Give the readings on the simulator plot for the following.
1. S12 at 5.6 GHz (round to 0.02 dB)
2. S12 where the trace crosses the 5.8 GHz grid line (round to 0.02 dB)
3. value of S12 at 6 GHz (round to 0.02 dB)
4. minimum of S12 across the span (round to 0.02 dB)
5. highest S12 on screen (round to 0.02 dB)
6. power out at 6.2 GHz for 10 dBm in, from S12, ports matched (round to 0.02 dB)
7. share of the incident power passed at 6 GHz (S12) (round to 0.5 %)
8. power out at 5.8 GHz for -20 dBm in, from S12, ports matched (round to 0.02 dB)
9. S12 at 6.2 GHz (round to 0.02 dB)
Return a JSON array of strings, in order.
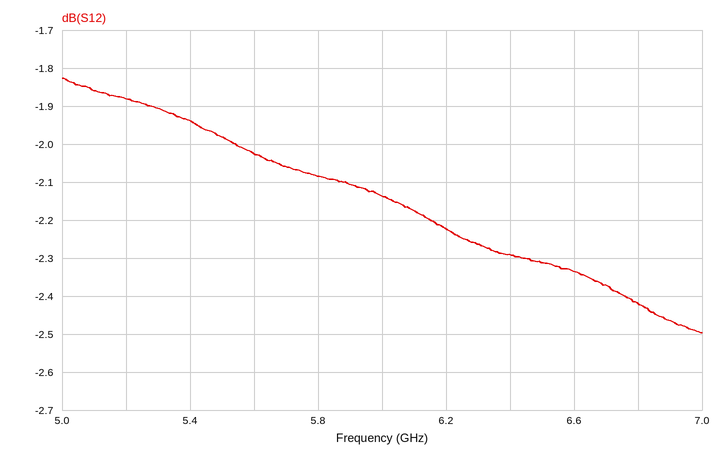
["-2.02 dB", "-2.08 dB", "-2.14 dB", "-2.50 dB", "-1.82 dB", "7.78 dBm", "61.0 %", "-22.08 dBm", "-2.22 dB"]
